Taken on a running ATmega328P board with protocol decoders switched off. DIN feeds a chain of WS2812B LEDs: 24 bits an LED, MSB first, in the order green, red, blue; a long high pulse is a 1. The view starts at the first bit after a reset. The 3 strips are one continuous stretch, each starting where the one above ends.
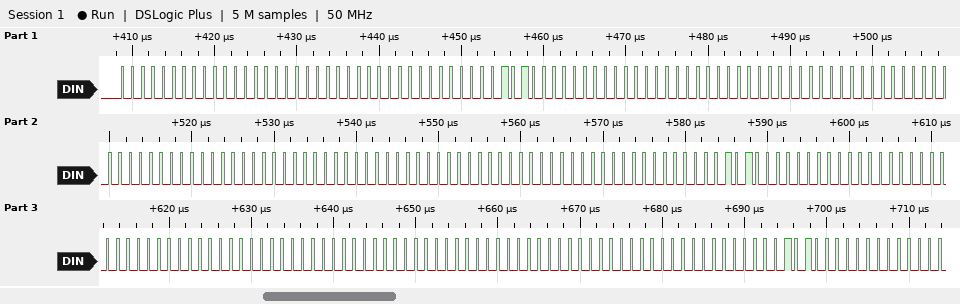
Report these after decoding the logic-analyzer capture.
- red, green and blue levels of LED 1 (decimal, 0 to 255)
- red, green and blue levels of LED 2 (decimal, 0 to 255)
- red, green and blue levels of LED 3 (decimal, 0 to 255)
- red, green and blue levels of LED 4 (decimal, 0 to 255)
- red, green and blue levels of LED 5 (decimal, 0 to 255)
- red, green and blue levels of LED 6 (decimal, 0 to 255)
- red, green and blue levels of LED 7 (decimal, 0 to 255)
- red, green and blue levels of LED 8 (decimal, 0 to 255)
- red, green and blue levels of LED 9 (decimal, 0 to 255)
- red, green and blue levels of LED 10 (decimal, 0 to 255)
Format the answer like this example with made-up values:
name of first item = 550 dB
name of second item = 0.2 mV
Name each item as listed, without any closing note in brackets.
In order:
red, green and blue levels of LED 1 = 0, 0, 0
red, green and blue levels of LED 2 = 5, 0, 0
red, green and blue levels of LED 3 = 0, 0, 0
red, green and blue levels of LED 4 = 0, 0, 0
red, green and blue levels of LED 5 = 0, 0, 0
red, green and blue levels of LED 6 = 0, 0, 5
red, green and blue levels of LED 7 = 0, 0, 0
red, green and blue levels of LED 8 = 0, 0, 0
red, green and blue levels of LED 9 = 0, 0, 0
red, green and blue levels of LED 10 = 5, 0, 0
